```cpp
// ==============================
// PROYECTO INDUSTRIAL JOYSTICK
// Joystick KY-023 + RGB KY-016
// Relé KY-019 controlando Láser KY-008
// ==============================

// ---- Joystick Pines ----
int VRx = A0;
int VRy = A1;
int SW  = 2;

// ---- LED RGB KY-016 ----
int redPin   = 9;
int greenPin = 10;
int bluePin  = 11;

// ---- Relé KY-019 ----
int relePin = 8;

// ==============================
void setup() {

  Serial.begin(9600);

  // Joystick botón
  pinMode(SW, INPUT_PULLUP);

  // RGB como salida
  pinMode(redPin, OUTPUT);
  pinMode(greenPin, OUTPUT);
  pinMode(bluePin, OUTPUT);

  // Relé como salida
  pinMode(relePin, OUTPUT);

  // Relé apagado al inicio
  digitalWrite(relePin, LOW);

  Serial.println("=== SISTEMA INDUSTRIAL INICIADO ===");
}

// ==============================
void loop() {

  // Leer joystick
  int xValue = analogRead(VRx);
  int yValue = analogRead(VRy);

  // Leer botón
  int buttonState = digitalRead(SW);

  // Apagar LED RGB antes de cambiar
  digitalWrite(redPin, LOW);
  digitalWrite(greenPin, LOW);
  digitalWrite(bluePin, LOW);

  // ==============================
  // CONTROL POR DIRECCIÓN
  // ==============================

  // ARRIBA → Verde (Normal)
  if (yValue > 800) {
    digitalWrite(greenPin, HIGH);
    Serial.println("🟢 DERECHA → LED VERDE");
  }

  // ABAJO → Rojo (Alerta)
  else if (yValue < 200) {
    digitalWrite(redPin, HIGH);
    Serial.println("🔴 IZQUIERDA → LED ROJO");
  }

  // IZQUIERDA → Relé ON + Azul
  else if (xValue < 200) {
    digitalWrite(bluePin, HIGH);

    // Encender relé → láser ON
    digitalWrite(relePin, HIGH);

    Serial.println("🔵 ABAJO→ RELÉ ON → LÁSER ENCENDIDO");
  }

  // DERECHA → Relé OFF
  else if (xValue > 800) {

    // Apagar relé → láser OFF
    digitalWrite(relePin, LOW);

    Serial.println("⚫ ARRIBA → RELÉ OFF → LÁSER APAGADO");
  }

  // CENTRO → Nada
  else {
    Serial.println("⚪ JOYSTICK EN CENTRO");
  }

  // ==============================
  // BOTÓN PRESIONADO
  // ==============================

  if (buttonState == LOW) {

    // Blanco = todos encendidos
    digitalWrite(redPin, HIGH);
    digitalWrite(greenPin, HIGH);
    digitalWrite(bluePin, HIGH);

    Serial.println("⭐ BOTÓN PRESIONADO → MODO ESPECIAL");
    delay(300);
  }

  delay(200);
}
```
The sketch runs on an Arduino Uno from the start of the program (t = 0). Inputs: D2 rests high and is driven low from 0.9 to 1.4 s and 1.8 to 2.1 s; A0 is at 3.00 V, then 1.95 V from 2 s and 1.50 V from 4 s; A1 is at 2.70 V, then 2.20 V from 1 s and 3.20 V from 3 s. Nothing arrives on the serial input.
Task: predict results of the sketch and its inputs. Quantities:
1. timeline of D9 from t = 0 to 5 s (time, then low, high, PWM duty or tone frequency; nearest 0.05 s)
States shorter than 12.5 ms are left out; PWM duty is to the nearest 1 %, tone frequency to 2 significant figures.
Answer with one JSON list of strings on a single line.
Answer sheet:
["0 s low; 1 s high; 1.5 s low; 1.9 s high; 2.4 s low"]
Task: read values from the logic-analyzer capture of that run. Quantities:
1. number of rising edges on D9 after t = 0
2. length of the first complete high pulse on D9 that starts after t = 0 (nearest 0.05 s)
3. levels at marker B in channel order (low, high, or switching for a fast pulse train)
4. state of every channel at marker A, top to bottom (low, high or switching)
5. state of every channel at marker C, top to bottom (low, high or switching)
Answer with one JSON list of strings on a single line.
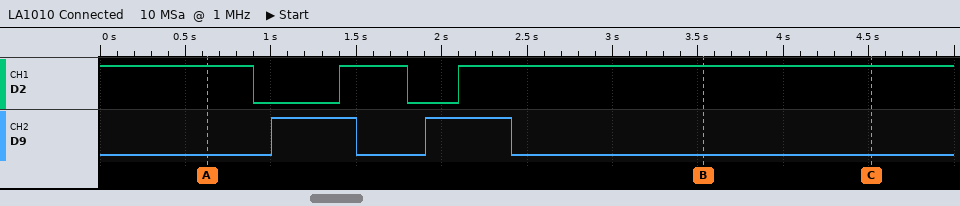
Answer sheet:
["2", "0.50 s", "D2 high, D9 low", "D2 high, D9 low", "D2 high, D9 low"]
